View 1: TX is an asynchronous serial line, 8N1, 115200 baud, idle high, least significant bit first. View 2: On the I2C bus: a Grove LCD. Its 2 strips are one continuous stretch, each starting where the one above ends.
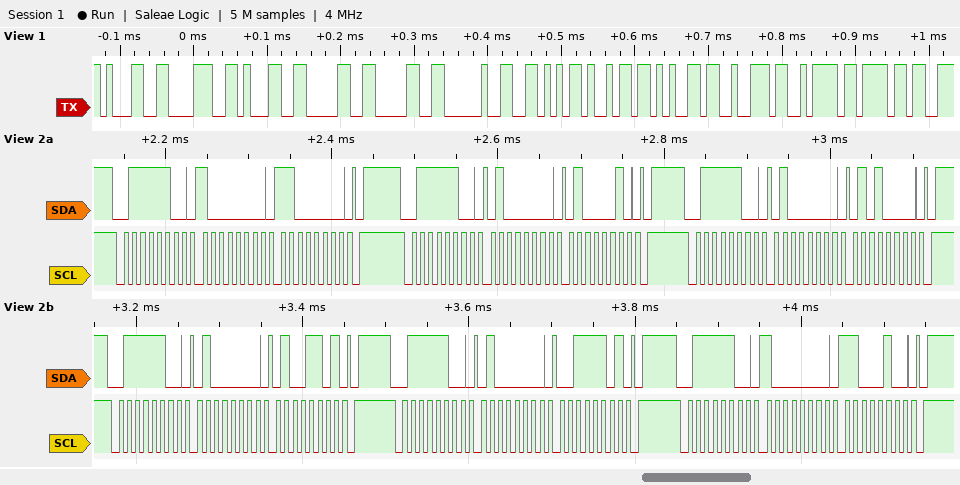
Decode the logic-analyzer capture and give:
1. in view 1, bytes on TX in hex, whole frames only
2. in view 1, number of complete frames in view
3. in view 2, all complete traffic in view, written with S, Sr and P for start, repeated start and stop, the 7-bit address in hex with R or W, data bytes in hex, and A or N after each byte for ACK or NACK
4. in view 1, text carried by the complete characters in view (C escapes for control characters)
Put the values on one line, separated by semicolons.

31 38 31 30 30 20 56 69 65 72 7A 6F; 12; S 3EW A 80 A C0 A P S 3EW A 40 A 42 A P S 3EW A 40 A 50 A P S 3EW A 40 A 4D A P S 3EW A 40 A 3D A P S 3EW A 80 A C4 A P; "18100 Vierzo"
